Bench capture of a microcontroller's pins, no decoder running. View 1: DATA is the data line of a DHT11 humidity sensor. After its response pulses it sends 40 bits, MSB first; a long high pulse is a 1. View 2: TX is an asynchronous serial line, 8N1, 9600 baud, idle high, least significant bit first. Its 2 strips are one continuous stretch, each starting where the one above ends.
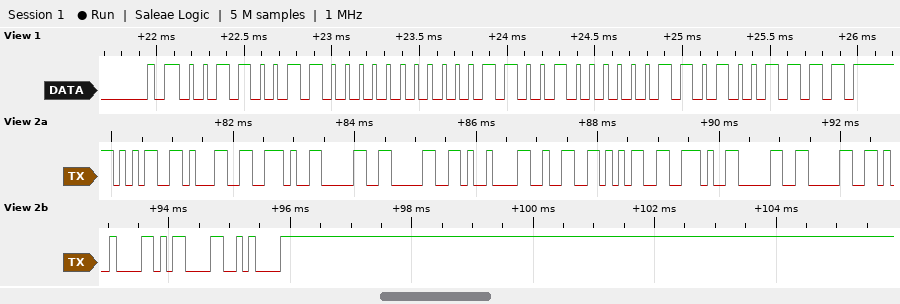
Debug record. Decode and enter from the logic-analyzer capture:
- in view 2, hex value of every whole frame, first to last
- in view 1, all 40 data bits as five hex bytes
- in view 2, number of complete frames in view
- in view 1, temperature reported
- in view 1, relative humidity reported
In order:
35 31 2E 30 30 09 32 35 2E 30 30 09 0D 0A
33 00 19 03 4F
14
25.3 °C
51 %
